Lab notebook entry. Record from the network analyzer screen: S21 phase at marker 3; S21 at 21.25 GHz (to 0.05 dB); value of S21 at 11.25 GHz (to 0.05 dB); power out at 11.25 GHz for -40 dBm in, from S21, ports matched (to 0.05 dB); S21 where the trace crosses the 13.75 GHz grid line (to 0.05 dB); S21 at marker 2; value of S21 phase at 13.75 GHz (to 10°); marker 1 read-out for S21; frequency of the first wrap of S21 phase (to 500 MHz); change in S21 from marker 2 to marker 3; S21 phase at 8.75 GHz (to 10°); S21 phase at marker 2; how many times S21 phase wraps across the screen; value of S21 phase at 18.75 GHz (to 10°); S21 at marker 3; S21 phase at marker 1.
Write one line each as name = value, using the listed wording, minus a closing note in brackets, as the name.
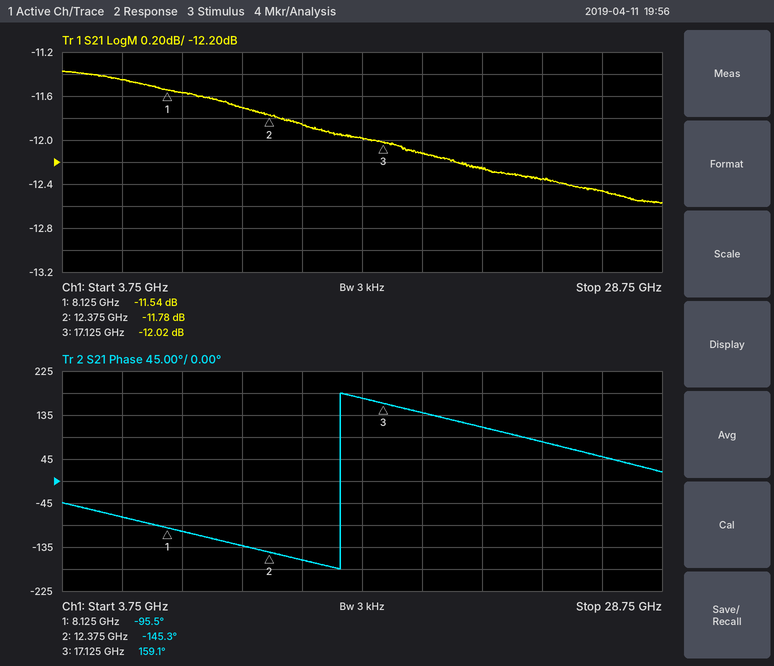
S21 phase at marker 3 = 159.1°
S21 at 21.25 GHz = -12.25 dB
value of S21 at 11.25 GHz = -11.70 dB
power out at 11.25 GHz for -40 dBm in, from S21, ports matched = -51.70 dBm
S21 where the trace crosses the 13.75 GHz grid line = -11.85 dB
S21 at marker 2 = -11.78 dB
value of S21 phase at 13.75 GHz = -160°
marker 1 read-out for S21 = -11.54 dB
frequency of the first wrap of S21 phase = 15.5 GHz
change in S21 from marker 2 to marker 3 = -0.24 dB
S21 phase at 8.75 GHz = -100°
S21 phase at marker 2 = -145.3°
how many times S21 phase wraps across the screen = 1
value of S21 phase at 18.75 GHz = 140°
S21 at marker 3 = -12.02 dB
S21 phase at marker 1 = -95.5°
